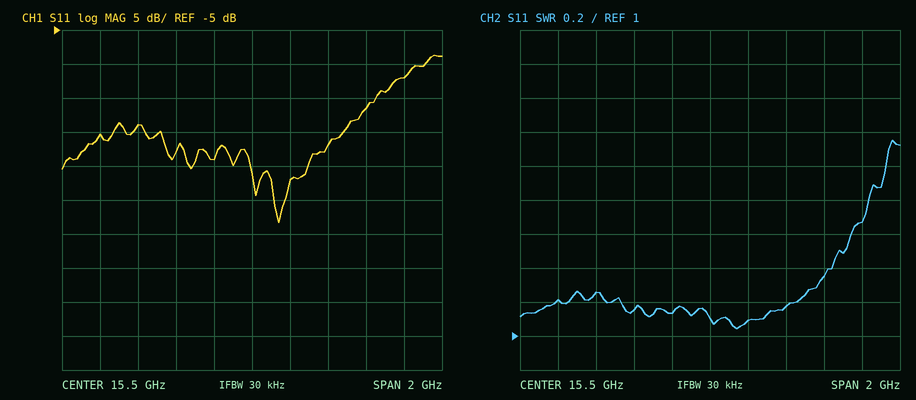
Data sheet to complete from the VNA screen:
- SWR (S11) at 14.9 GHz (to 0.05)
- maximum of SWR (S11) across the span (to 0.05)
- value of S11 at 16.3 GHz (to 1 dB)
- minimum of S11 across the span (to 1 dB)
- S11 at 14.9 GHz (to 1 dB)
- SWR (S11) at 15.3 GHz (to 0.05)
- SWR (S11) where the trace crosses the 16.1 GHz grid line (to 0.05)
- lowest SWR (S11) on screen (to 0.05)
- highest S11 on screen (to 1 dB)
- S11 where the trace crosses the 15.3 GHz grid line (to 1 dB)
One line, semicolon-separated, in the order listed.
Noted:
1.25; 2.15; -12 dB; -33 dB; -19 dB; 1.15; 1.35; 1.05; -9 dB; -24 dB
